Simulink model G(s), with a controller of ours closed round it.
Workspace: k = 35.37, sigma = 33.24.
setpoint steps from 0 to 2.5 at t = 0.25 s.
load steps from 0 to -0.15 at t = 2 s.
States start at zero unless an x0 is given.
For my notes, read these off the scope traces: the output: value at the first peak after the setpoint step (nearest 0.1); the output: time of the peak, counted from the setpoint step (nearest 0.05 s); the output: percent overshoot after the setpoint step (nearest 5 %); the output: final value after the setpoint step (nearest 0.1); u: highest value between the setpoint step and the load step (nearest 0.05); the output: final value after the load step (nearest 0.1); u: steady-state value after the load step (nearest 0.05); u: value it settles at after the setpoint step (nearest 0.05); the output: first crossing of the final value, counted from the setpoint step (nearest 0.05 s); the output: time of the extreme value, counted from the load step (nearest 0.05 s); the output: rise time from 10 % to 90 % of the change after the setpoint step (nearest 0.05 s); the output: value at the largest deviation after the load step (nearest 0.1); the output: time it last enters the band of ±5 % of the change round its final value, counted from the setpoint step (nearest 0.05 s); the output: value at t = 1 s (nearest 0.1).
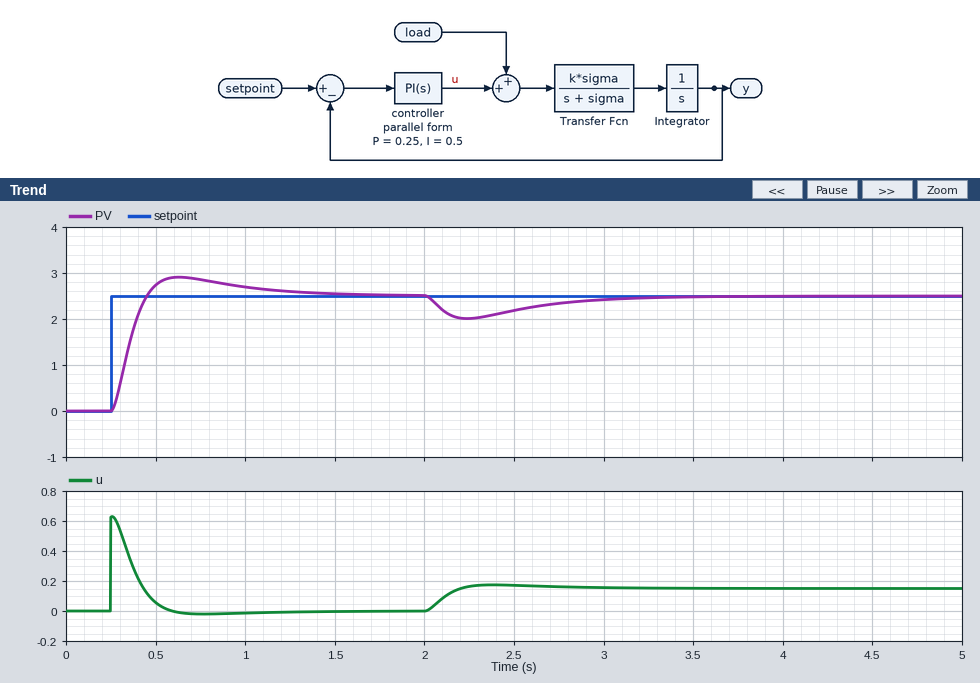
2.9
0.40 s
15 %
2.5
0.65
2.5
0.15
0.00
0.20 s
0.25 s
0.15 s
2.0
0.90 s
2.7
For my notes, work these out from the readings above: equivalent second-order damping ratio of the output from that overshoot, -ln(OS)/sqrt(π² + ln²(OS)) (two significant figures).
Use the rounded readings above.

0.52
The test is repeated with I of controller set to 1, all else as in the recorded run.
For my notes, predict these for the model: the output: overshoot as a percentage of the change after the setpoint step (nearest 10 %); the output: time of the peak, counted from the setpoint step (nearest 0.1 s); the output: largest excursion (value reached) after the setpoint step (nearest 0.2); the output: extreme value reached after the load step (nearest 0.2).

30 %
0.3 s
3.2
2.0
